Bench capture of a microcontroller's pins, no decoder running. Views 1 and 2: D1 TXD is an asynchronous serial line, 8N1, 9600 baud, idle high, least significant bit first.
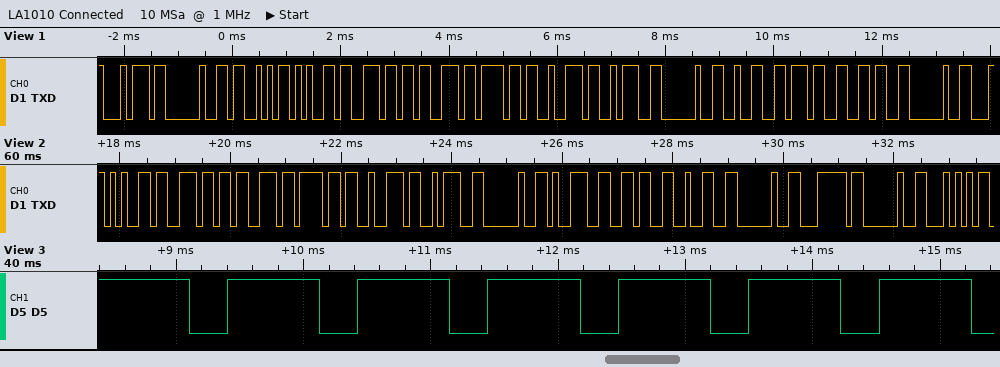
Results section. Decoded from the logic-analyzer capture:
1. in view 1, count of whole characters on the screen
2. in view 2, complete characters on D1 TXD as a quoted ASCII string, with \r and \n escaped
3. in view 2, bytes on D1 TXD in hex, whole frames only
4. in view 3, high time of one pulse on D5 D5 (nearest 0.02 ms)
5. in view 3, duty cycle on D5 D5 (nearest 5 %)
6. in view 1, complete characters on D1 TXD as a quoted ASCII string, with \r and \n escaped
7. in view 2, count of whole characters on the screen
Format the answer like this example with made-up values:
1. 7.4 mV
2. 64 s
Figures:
1. 14
2. "ensor: 962 | T"
3. 65 6E 73 6F 72 3A 20 39 36 32 20 7C 20 54
4. 0.72 ms
5. 70 %
6. "t Sensor: 276 "
7. 14
